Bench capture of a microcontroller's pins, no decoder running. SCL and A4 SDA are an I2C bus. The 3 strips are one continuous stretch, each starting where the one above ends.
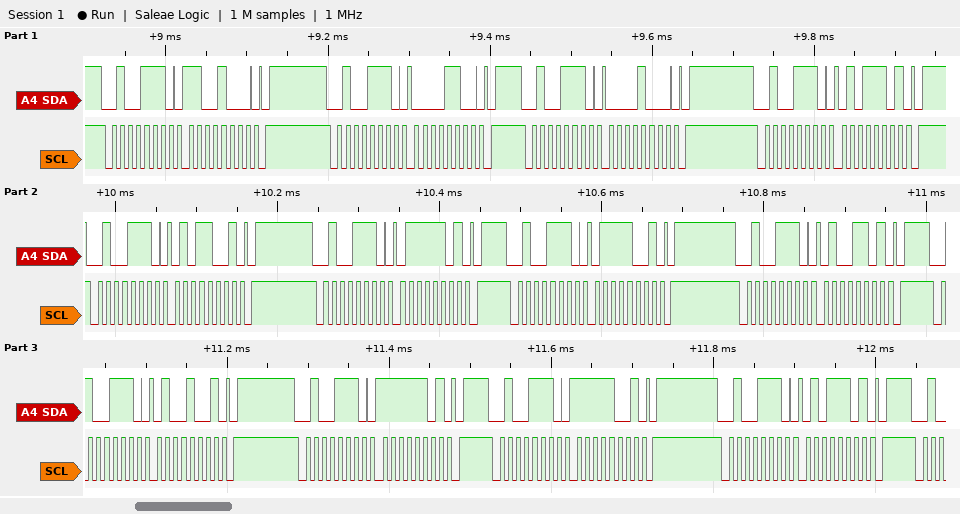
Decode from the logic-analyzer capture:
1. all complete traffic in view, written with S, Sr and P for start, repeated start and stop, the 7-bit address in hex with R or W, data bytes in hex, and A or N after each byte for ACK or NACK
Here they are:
S 27W A C8 A P S 27W A 0C A P S 27W A 08 A P S 27W A 5D A P S 27W A 59 A P S 27W A 7D A P S 27W A 79 A P S 27W A 4D A P S 27W A 49 A P S 27W A FD A P S 27W A F9 A P S 27W A 5D A P
